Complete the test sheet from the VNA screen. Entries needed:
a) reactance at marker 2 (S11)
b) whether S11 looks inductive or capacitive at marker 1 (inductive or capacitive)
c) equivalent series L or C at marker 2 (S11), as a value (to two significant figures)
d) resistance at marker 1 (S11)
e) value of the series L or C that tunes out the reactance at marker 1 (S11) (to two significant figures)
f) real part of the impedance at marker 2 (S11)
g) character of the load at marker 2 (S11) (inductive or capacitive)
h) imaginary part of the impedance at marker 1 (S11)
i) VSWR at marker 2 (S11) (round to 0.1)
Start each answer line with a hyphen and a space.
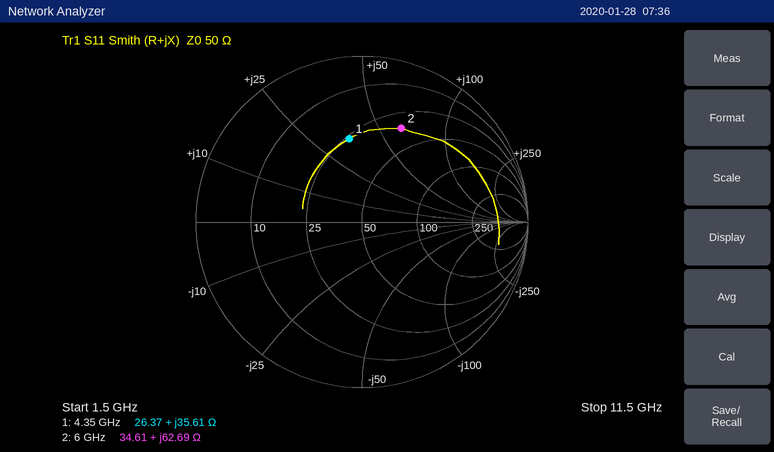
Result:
- +62.69 Ω
- inductive
- 1.7 nH
- 26.37 Ω
- 1.0 pF
- 34.61 Ω
- inductive
- +35.61 Ω
- 4.2
